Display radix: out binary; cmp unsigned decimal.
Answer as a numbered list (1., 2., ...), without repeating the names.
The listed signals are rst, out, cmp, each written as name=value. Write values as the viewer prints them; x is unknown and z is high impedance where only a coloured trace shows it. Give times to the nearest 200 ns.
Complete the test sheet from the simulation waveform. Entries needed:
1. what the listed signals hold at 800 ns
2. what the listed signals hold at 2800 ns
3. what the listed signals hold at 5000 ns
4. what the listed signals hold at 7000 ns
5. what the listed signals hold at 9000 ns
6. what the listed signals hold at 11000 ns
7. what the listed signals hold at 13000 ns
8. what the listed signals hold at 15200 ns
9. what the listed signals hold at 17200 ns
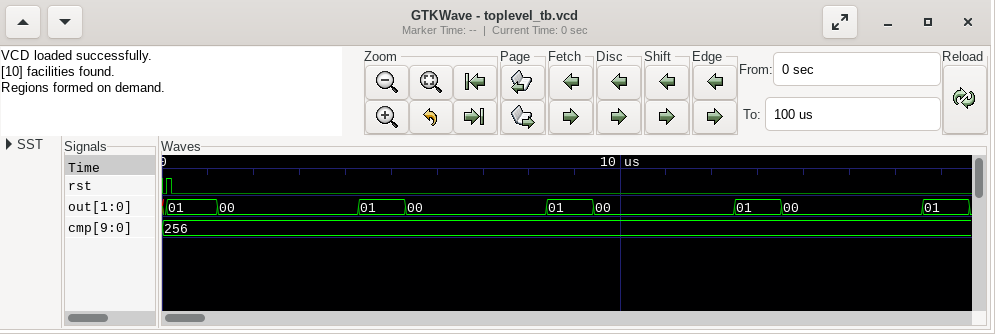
1. rst=0, out=01, cmp=256
2. rst=0, out=00, cmp=256
3. rst=0, out=01, cmp=256
4. rst=0, out=00, cmp=256
5. rst=0, out=01, cmp=256
6. rst=0, out=00, cmp=256
7. rst=0, out=01, cmp=256
8. rst=0, out=00, cmp=256
9. rst=0, out=01, cmp=256
